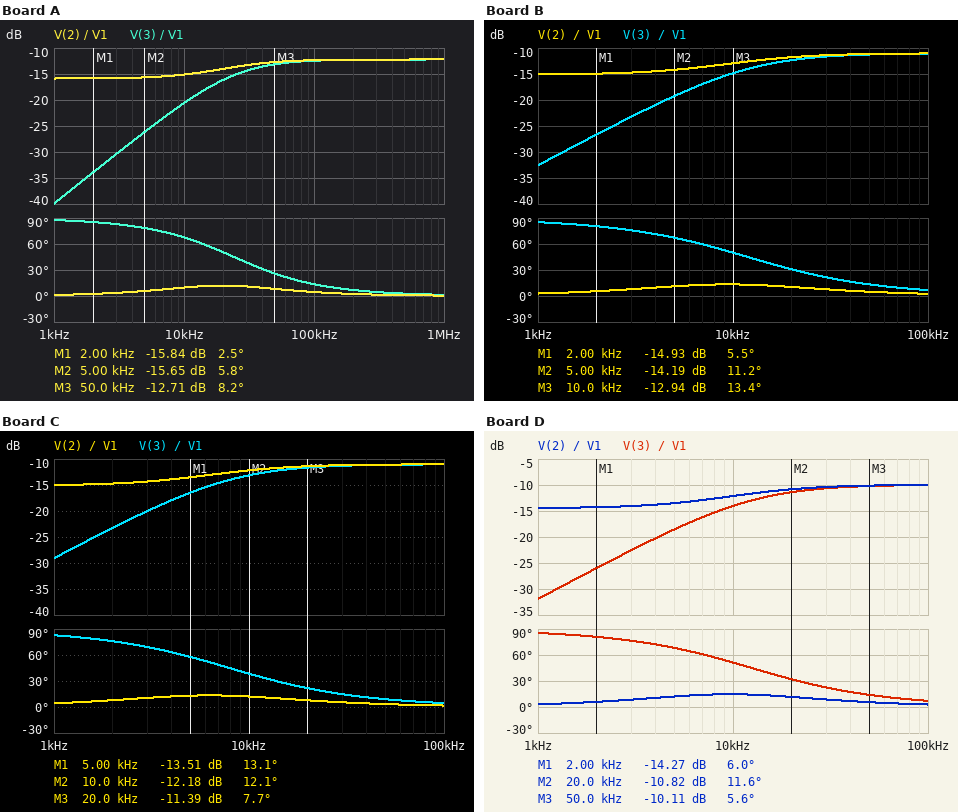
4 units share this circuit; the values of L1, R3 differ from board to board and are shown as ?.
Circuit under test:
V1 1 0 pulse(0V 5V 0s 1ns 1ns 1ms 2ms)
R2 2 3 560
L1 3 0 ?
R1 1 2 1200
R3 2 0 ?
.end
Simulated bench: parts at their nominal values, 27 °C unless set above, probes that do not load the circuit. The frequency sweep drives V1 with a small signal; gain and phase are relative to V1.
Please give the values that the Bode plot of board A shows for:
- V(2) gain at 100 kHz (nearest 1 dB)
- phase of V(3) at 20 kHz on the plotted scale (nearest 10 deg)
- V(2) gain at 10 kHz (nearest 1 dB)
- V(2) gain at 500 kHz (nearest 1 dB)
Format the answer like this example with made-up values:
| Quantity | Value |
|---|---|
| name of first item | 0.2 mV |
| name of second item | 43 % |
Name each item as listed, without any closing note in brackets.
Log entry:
| Quantity | Value |
|---|---|
| V(2) gain at 100 kHz | -12 dB |
| phase of V(3) at 20 kHz on the plotted scale | 50 deg |
| V(2) gain at 10 kHz | -15 dB |
| V(2) gain at 500 kHz | -12 dB |
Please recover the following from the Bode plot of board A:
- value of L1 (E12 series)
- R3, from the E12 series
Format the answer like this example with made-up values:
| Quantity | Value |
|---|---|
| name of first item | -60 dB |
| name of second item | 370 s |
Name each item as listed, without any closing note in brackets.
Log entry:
| Quantity | Value |
|---|---|
| value of L1 | 5.6 mH |
| R3, from the E12 series | 390 Ω |
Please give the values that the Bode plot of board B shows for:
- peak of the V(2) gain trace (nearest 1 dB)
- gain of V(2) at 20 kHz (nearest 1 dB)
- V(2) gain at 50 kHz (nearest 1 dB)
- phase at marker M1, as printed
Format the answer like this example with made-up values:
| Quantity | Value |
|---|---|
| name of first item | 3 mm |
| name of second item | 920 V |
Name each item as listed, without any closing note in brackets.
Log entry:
| Quantity | Value |
|---|---|
| peak of the V(2) gain trace | -11 dB |
| gain of V(2) at 20 kHz | -12 dB |
| V(2) gain at 50 kHz | -11 dB |
| phase at marker M1, as printed | 5.5 deg |
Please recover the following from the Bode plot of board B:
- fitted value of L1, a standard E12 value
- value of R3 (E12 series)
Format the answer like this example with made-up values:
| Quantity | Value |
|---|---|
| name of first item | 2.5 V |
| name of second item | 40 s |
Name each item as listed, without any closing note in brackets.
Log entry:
| Quantity | Value |
|---|---|
| fitted value of L1, a standard E12 value | 12 mH |
| value of R3 | 470 Ω |
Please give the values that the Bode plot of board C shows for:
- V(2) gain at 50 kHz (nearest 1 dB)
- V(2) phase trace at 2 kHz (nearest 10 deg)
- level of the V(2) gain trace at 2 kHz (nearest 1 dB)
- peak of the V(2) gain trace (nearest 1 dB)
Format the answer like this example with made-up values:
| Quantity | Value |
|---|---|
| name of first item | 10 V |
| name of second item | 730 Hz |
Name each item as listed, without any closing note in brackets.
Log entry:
| Quantity | Value |
|---|---|
| V(2) gain at 50 kHz | -11 dB |
| V(2) phase trace at 2 kHz | 10 deg |
| level of the V(2) gain trace at 2 kHz | -15 dB |
| peak of the V(2) gain trace | -11 dB |
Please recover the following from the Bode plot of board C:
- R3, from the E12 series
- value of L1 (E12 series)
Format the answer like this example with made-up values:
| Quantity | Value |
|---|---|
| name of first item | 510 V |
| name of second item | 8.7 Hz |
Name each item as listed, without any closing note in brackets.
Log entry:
| Quantity | Value |
|---|---|
| R3, from the E12 series | 470 Ω |
| value of L1 | 18 mH |
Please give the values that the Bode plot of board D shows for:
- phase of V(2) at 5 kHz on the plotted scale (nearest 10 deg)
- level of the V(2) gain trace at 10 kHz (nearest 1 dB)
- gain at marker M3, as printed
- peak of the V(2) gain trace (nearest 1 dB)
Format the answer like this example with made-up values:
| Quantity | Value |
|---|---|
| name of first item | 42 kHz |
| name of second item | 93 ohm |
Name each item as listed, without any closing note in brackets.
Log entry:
| Quantity | Value |
|---|---|
| phase of V(2) at 5 kHz on the plotted scale | 10 deg |
| level of the V(2) gain trace at 10 kHz | -12 dB |
| gain at marker M3, as printed | -10.11 dB |
| peak of the V(2) gain trace | -10 dB |
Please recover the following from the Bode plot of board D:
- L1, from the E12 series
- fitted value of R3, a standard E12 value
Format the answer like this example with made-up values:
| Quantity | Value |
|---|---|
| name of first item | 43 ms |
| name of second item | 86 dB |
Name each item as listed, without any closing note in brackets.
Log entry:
| Quantity | Value |
|---|---|
| L1, from the E12 series | 12 mH |
| fitted value of R3, a standard E12 value | 560 Ω |
